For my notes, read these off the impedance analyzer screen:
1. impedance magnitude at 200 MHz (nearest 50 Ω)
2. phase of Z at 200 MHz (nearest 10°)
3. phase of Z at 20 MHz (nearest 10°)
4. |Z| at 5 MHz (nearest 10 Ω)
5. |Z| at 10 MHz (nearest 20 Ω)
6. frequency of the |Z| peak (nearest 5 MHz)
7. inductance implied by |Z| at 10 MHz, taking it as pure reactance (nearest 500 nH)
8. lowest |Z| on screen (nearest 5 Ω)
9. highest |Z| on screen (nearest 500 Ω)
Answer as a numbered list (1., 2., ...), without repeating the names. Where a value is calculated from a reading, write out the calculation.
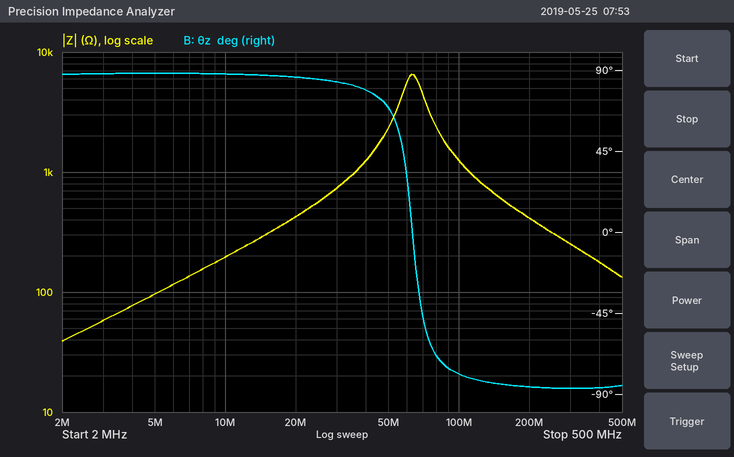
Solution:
1. 400 Ω
2. -90°
3. 90°
4. 100 Ω
5. 200 Ω
6. 65 MHz
7. L = 200 Ω/(2π × 10 MHz) ≈ 3.18 µH, so 3.0 µH to the nearest 500 nH
8. 40 Ω
9. 6.5 kΩ
